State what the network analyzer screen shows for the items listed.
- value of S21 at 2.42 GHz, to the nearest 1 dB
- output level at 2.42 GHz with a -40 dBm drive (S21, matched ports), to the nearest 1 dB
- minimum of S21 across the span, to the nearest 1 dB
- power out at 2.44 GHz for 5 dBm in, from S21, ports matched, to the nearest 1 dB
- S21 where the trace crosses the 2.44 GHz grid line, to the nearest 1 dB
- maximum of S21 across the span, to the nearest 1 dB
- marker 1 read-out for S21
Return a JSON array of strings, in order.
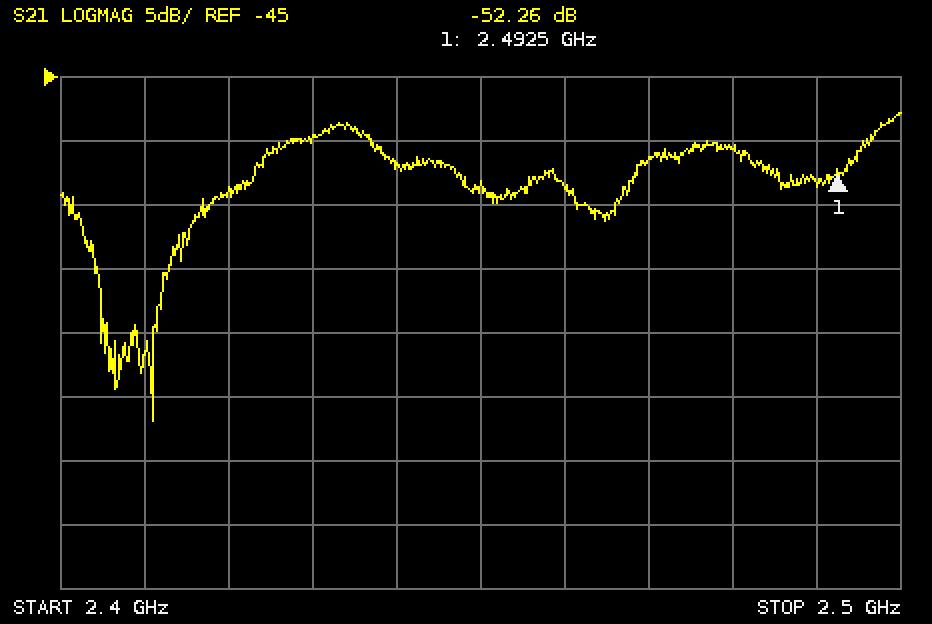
["-54 dB", "-94 dBm", "-72 dB", "-47 dBm", "-52 dB", "-48 dB", "-52.26 dB"]
